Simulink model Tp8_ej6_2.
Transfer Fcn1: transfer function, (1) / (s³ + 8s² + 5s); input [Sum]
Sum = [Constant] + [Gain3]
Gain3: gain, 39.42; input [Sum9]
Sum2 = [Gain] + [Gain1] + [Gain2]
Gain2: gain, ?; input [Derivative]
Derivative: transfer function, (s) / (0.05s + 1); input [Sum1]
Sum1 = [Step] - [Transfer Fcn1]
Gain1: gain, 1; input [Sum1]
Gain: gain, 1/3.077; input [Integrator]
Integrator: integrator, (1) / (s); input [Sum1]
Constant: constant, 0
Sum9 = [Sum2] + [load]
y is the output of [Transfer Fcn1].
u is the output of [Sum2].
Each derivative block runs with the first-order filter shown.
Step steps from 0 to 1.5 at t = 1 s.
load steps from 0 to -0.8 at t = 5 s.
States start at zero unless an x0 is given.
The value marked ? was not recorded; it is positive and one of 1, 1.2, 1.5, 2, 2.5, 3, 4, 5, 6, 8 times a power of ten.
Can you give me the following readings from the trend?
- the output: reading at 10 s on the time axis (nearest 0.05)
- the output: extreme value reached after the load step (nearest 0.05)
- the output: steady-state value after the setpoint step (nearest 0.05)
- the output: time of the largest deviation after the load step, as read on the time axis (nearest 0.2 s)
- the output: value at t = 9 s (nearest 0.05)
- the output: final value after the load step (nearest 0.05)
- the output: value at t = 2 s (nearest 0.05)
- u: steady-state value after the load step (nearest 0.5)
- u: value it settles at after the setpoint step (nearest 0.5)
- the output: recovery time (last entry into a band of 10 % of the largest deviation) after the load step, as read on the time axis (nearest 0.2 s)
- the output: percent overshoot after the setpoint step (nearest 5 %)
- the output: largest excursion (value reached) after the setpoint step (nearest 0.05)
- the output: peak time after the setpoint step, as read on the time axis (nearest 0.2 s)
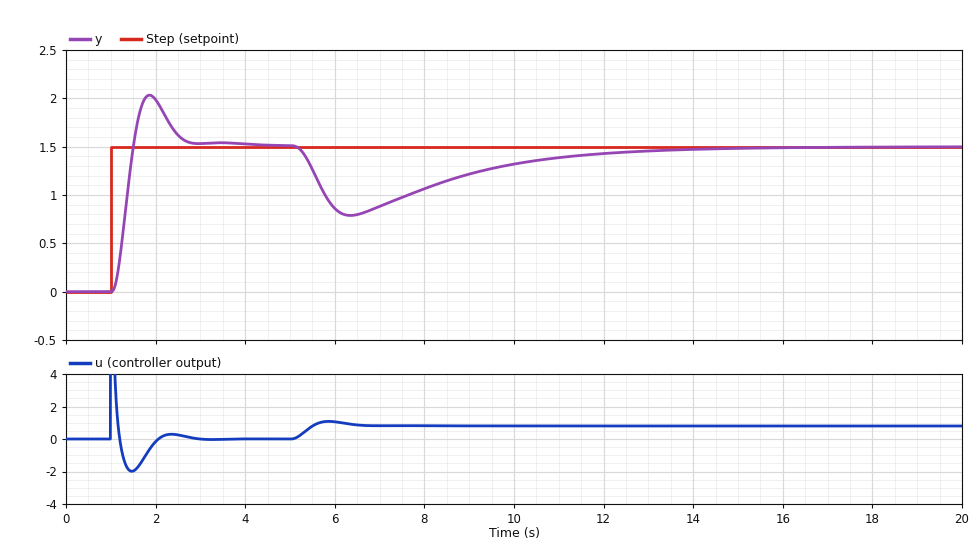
1.30
0.80
1.50
6.4 s
1.20
1.50
2.00
1.0
0.0
12.0 s
35 %
2.05
1.8 s
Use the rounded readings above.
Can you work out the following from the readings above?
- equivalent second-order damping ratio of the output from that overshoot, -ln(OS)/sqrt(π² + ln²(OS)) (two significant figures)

0.32
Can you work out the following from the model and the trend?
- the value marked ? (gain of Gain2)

0.6
